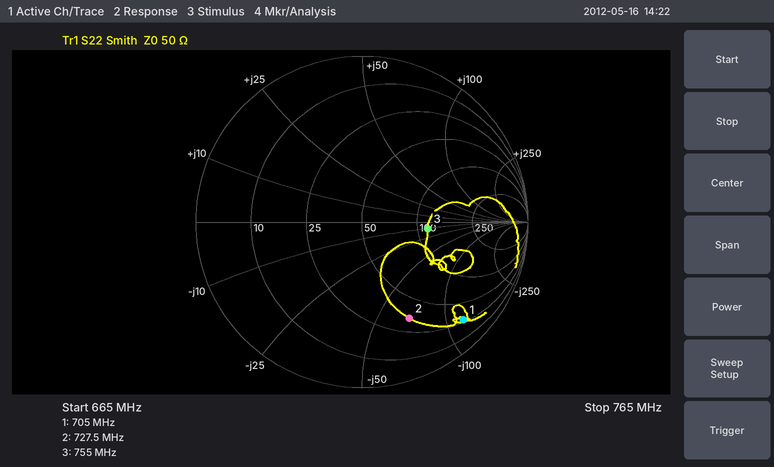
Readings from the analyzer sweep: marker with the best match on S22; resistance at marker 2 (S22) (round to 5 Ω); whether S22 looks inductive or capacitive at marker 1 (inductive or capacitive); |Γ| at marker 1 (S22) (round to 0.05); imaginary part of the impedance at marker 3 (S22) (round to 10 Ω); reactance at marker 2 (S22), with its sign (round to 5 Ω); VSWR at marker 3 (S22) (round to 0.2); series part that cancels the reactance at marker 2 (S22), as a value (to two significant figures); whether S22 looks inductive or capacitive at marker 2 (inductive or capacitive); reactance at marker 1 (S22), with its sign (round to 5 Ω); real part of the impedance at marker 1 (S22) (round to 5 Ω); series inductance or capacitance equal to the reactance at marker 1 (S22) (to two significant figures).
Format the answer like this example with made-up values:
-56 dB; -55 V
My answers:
marker 3; 35 Ω; capacitive; 0.85; -10 Ω; -70 Ω; 2.4; 15 nH; capacitive; -120 Ω; 30 Ω; 1.9 pF
